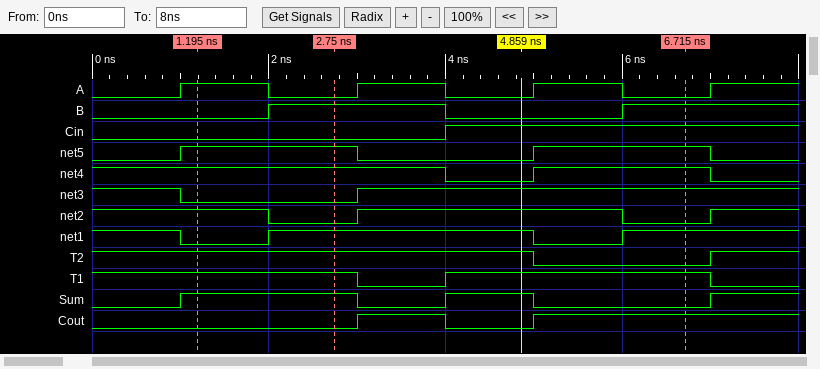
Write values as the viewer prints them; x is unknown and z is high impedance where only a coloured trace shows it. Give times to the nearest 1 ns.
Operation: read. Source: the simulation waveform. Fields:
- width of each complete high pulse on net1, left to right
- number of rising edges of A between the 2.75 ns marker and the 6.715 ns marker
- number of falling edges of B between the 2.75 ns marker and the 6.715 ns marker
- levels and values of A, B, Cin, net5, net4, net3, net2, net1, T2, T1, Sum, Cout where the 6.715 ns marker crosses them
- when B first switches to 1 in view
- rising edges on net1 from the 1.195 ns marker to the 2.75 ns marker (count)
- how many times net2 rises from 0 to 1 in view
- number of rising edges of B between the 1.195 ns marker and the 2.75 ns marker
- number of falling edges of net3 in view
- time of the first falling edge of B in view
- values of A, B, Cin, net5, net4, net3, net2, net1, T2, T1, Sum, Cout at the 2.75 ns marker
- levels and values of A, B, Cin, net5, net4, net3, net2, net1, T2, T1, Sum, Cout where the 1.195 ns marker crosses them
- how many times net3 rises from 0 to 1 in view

3 ns
2
1
A=0, B=1, Cin=1, net5=1, net4=1, net3=1, net2=0, net1=1, T2=0, T1=1, Sum=0, Cout=1
2 ns
1
2
1
1
4 ns
A=0, B=1, Cin=0, net5=1, net4=1, net3=0, net2=0, net1=1, T2=1, T1=1, Sum=1, Cout=0
A=1, B=0, Cin=0, net5=1, net4=1, net3=0, net2=1, net1=0, T2=1, T1=1, Sum=1, Cout=0
1
